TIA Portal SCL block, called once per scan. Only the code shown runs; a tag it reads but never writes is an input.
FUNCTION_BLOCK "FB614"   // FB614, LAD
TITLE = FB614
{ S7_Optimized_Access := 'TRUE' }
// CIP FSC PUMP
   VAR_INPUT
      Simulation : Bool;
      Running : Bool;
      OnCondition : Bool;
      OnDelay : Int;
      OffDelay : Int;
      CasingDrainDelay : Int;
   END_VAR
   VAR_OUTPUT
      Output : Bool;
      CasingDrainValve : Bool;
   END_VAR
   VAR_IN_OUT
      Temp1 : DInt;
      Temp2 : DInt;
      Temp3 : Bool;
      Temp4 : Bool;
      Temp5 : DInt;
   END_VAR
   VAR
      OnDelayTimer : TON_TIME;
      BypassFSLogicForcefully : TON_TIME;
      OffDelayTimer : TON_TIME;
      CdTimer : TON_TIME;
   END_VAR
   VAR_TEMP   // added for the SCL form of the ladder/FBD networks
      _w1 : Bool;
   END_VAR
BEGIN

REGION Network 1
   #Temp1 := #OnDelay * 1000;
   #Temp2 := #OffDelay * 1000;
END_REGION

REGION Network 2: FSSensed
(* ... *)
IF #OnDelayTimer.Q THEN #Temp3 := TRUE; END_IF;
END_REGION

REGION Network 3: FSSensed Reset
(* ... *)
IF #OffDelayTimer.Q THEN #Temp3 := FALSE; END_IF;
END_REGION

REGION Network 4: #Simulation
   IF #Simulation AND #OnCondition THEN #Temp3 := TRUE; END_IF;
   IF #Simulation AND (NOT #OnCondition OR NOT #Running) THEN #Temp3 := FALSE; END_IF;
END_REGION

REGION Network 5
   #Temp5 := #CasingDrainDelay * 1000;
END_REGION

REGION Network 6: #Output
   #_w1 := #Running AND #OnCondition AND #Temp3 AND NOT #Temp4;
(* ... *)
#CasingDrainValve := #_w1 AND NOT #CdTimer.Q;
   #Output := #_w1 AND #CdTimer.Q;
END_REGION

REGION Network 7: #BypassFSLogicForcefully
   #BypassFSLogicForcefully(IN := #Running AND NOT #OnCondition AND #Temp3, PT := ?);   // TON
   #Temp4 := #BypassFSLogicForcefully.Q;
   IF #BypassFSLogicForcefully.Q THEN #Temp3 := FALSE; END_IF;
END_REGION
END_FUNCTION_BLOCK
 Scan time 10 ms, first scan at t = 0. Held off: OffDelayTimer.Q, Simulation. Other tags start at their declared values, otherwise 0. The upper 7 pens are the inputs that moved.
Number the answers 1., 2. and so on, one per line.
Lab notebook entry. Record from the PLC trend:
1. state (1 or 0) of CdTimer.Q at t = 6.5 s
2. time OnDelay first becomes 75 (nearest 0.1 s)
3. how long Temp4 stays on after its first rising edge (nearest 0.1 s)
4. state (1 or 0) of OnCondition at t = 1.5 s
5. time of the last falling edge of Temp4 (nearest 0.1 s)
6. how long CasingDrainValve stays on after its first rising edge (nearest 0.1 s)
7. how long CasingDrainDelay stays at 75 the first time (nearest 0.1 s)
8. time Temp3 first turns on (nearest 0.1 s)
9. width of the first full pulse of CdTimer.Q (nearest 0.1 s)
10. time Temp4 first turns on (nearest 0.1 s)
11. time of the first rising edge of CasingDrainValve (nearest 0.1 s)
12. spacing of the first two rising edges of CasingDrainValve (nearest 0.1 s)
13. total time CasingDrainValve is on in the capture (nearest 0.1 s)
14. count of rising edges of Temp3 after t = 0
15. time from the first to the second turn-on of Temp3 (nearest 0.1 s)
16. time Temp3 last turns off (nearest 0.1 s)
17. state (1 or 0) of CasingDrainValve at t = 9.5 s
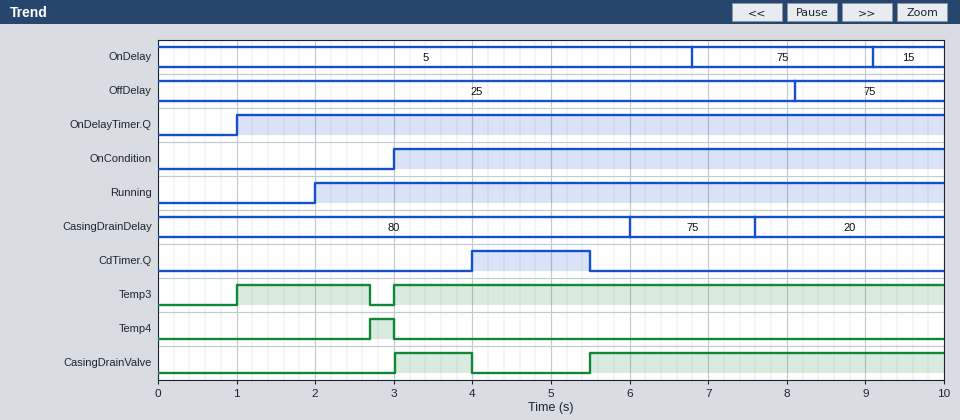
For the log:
1. 0
2. 6.8 s
3. 0.3 s
4. 0
5. 3.0 s
6. 1.0 s
7. 1.6 s
8. 1.0 s
9. 1.5 s
10. 2.7 s
11. 3.0 s
12. 2.5 s
13. 5.5 s
14. 2
15. 2.0 s
16. 2.7 s
17. 1
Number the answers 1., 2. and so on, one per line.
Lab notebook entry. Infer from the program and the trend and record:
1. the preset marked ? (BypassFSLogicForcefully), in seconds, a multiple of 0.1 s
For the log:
1. 0.7 s
